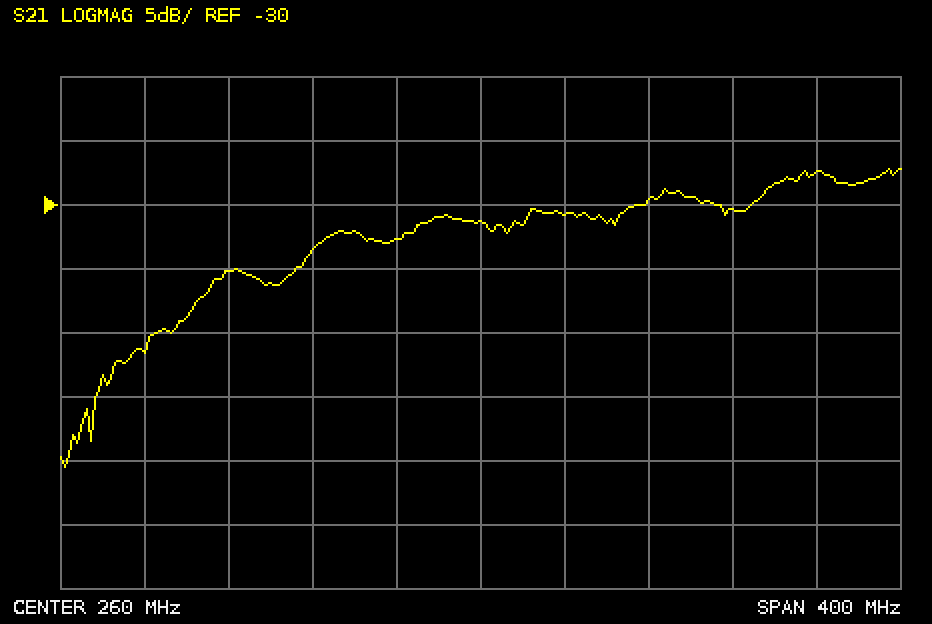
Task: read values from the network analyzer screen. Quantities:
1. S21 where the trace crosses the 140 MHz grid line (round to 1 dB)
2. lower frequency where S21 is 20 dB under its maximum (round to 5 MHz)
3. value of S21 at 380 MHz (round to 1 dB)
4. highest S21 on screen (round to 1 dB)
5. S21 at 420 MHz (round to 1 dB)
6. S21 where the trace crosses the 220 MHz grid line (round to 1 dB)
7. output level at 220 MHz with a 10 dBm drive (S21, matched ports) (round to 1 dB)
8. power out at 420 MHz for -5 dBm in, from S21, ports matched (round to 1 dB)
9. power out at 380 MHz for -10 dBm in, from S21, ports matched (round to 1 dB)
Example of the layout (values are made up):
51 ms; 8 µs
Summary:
-35 dB; 75 MHz; -30 dB; -27 dB; -27 dB; -33 dB; -23 dBm; -32 dBm; -40 dBm
